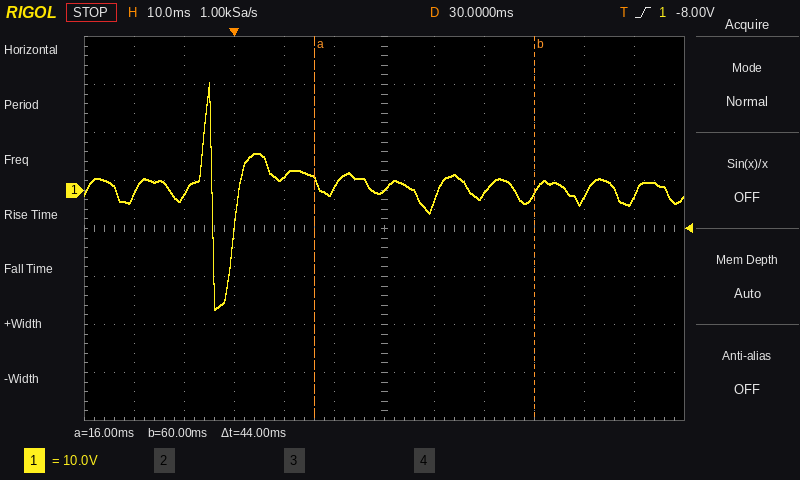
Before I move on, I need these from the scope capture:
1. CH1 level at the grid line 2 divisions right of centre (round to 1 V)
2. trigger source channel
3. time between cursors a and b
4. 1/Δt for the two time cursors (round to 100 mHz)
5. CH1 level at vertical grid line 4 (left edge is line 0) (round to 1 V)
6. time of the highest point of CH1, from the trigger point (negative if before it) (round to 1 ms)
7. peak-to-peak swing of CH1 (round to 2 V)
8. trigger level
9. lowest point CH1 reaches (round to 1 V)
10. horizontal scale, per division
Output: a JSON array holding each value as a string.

["-1 V", "CH1", "44 ms", "22.7 Hz", "3 V", "-5 ms", "48 V", "-8.00 V", "-25 V", "10 ms"]
